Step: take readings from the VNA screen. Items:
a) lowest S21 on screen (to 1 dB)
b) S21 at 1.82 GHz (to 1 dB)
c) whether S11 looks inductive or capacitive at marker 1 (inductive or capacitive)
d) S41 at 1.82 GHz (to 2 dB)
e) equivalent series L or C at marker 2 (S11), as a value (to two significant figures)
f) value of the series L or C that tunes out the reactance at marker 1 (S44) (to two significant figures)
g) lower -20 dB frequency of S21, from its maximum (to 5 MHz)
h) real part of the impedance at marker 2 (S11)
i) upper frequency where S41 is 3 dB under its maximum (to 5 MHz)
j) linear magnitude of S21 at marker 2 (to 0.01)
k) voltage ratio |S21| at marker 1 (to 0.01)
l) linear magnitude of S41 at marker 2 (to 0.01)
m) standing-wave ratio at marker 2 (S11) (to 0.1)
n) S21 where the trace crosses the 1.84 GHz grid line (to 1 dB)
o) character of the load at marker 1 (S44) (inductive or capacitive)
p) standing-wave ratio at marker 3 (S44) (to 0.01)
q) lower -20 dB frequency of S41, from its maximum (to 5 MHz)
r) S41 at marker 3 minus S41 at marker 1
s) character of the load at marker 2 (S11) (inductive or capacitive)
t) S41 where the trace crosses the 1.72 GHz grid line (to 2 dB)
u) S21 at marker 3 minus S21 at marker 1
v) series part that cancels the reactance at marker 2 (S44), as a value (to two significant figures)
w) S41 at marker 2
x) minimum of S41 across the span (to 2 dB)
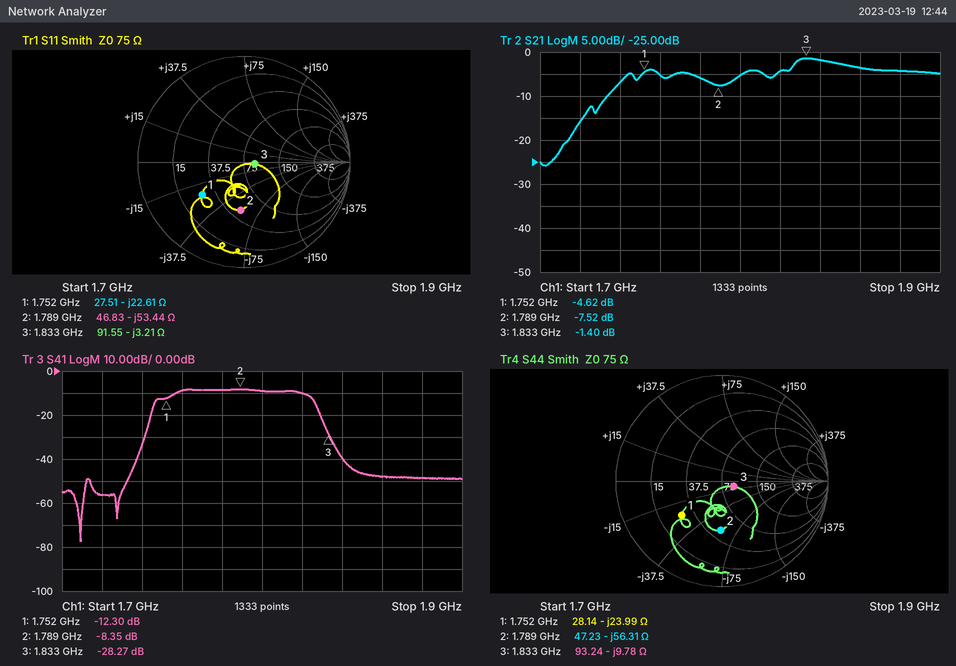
-26 dB
-4 dB
capacitive
-10 dB
1.7 pF
2.2 nH
1.710 GHz
46.83 Ω
1.825 GHz
0.42
0.59
0.38
2.7
-2 dB
capacitive
1.28
1.740 GHz
-15.97 dB
capacitive
-56 dB
3.22 dB
5.0 nH
-8.35 dB
-78 dB
